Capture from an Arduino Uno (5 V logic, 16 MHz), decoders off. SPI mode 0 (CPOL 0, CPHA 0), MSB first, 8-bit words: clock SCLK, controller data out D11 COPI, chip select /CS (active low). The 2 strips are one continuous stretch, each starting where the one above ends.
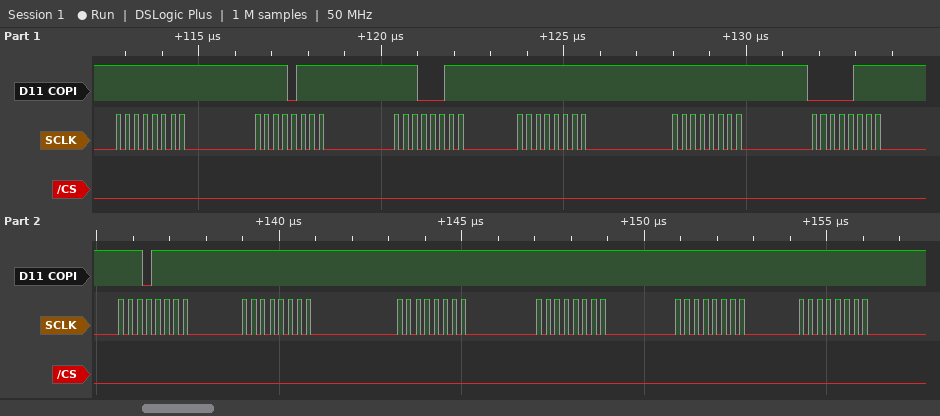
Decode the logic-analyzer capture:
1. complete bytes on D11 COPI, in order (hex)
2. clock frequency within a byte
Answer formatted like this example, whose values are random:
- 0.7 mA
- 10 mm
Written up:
- 0xFF 0xF7 0xE3 0xFF 0xFF 0x07 0xEF 0xFF 0xFF 0xFF 0xFF 0xFF
- 4 MHz
